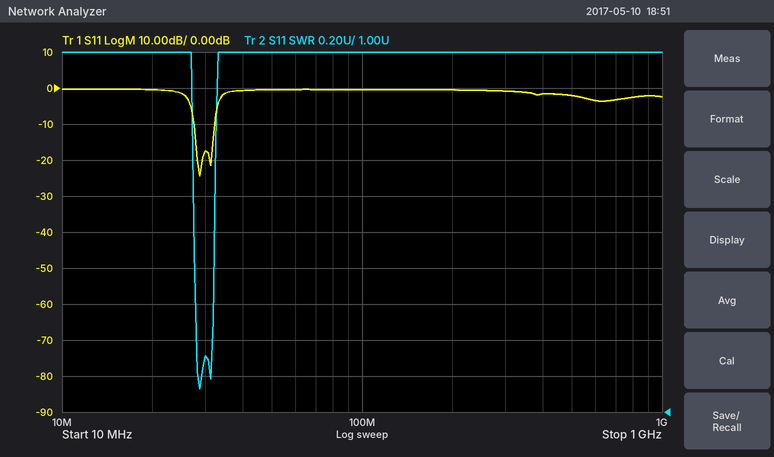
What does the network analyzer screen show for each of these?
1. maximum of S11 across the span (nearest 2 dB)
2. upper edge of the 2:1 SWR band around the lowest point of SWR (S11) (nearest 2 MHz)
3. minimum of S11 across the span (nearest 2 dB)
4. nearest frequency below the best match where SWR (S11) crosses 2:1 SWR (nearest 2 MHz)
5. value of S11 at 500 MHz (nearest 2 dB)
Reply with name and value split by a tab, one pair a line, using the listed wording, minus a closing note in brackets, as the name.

maximum of S11 across the span	0 dB
upper edge of the 2:1 SWR band around the lowest point of SWR (S11)	32 MHz
minimum of S11 across the span	-24 dB
nearest frequency below the best match where SWR (S11) crosses 2:1 SWR	28 MHz
value of S11 at 500 MHz	-2 dB
